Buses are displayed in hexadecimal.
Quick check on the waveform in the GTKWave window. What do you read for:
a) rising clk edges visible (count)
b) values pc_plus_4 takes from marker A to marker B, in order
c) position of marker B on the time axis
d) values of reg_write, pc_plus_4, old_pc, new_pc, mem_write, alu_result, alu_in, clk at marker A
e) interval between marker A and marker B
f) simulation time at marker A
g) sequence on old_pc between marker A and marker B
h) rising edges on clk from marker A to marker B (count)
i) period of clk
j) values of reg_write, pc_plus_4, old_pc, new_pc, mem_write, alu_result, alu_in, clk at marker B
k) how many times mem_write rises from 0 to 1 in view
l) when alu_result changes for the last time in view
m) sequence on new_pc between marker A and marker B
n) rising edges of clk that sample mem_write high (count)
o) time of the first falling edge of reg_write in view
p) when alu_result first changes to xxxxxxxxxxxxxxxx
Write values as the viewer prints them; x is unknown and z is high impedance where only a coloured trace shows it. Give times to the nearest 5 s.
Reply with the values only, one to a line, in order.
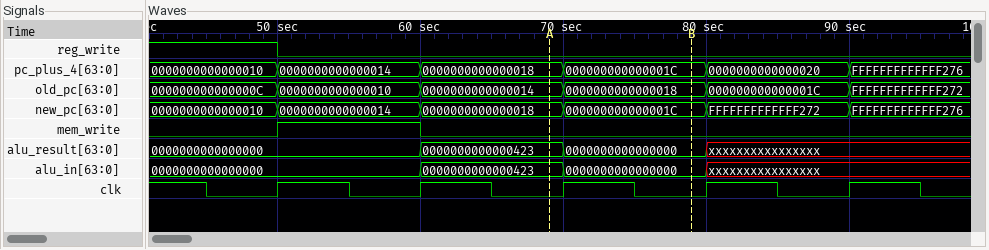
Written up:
5
0000000000000018, 000000000000001C
80 s
reg_write=0, pc_plus_4=0000000000000018, old_pc=0000000000000014, new_pc=0000000000000018, mem_write=0, alu_result=0000000000000423, alu_in=0000000000000423, clk=0
10 s
70 s
0000000000000014, 0000000000000018
1
10 s
reg_write=0, pc_plus_4=000000000000001C, old_pc=0000000000000018, new_pc=000000000000001C, mem_write=0, alu_result=0000000000000000, alu_in=0000000000000000, clk=0
1
80 s
0000000000000018, 000000000000001C
1
50 s
80 s
